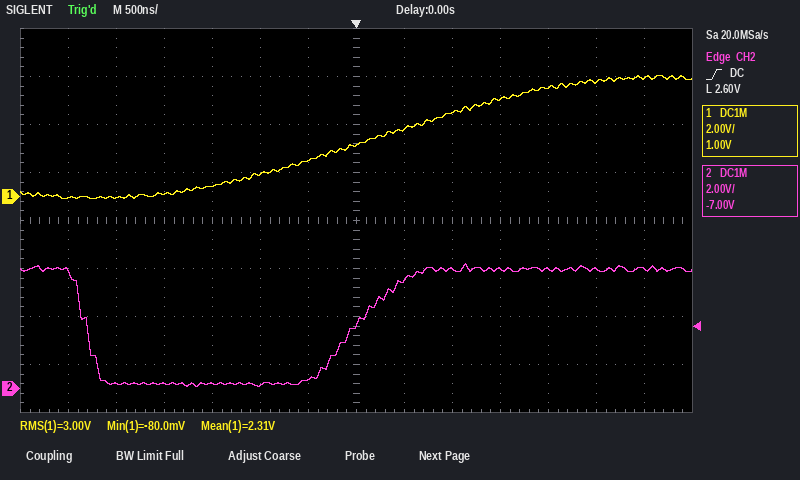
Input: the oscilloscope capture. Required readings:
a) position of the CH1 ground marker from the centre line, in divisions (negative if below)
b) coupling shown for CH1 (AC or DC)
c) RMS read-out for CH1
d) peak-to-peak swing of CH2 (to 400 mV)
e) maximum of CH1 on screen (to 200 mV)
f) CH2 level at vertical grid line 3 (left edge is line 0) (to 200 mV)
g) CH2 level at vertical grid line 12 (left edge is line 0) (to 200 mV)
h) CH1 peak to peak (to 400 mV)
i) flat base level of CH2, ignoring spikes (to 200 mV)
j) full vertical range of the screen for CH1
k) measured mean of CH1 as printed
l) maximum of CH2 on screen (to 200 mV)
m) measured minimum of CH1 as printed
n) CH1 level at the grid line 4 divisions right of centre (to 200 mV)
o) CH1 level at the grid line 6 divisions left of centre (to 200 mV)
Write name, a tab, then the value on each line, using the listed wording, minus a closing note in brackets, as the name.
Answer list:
position of the CH1 ground marker from the centre line, in divisions	+0.5 div
coupling shown for CH1	DC
RMS read-out for CH1	3.00 V
peak-to-peak swing of CH2	5.2 V
maximum of CH1 on screen	5.0 V
CH2 level at vertical grid line 3 (left edge is line 0)	200 mV
CH2 level at vertical grid line 12 (left edge is line 0)	5.0 V
CH1 peak to peak	5.2 V
flat base level of CH2, ignoring spikes	200 mV
full vertical range of the screen for CH1	16 V
measured mean of CH1 as printed	2.31 V
maximum of CH2 on screen	5.2 V
measured minimum of CH1 as printed	-80.0 mV
CH1 level at the grid line 4 divisions right of centre	4.6 V
CH1 level at the grid line 6 divisions left of centre	0.0 V
